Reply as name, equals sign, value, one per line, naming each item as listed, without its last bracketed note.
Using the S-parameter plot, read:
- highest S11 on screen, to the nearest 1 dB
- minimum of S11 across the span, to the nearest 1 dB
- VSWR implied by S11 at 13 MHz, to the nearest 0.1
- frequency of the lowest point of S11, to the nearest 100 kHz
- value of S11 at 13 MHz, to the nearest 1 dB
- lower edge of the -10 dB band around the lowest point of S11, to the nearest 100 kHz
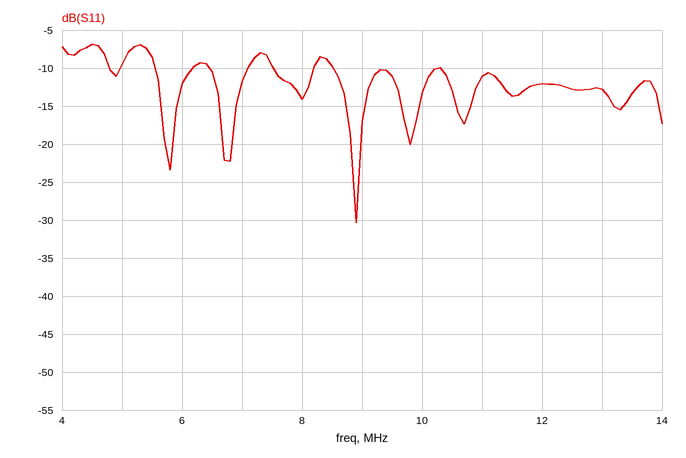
highest S11 on screen, to the nearest 1 dB = -7 dB
minimum of S11 across the span, to the nearest 1 dB = -30 dB
VSWR implied by S11 at 13 MHz, to the nearest 0.1 = 1.6
frequency of the lowest point of S11, to the nearest 100 kHz = 8.9 MHz
value of S11 at 13 MHz, to the nearest 1 dB = -13 dB
lower edge of the -10 dB band around the lowest point of S11, to the nearest 100 kHz = 8.5 MHz
